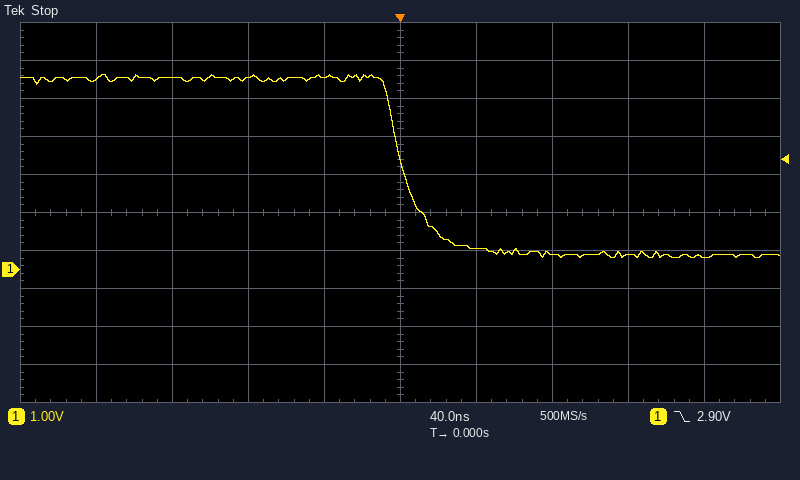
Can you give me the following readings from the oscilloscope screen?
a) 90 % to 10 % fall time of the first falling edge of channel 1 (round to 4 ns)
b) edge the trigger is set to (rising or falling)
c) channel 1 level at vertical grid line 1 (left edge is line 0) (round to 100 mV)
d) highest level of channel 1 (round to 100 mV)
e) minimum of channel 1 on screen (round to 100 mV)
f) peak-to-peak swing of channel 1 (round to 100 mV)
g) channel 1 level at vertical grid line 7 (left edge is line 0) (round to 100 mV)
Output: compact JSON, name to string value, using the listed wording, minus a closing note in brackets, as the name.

{"90 % to 10 % fall time of the first falling edge of channel 1": "28 ns", "edge the trigger is set to": "falling", "channel 1 level at vertical grid line 1 (left edge is line 0)": "5.0 V", "highest level of channel 1": "5.1 V", "minimum of channel 1 on screen": "300 mV", "peak-to-peak swing of channel 1": "4.8 V", "channel 1 level at vertical grid line 7 (left edge is line 0)": "400 mV"}
